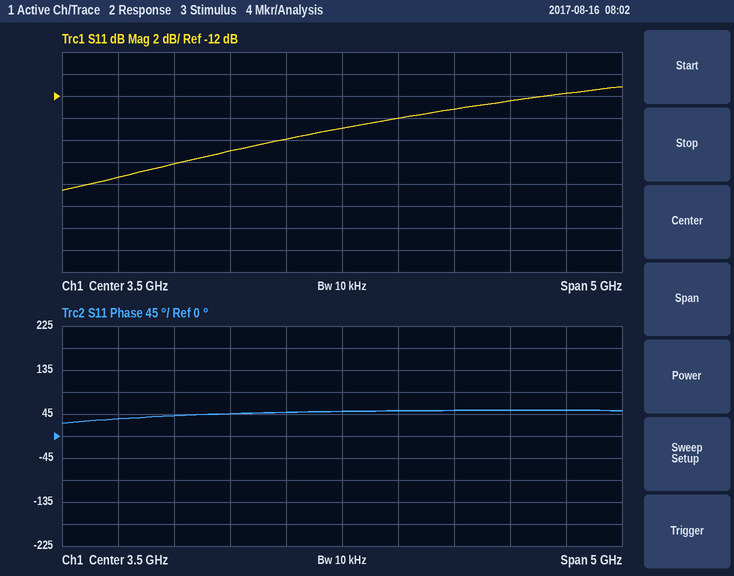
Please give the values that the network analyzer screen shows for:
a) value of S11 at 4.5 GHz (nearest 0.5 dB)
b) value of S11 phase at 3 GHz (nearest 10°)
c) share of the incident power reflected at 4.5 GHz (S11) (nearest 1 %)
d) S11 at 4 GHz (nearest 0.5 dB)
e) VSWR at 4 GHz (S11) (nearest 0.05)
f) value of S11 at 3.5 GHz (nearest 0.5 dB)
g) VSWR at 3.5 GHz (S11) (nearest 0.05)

-13.0 dB
50°
5 %
-14.0 dB
1.50
-15.0 dB
1.45
